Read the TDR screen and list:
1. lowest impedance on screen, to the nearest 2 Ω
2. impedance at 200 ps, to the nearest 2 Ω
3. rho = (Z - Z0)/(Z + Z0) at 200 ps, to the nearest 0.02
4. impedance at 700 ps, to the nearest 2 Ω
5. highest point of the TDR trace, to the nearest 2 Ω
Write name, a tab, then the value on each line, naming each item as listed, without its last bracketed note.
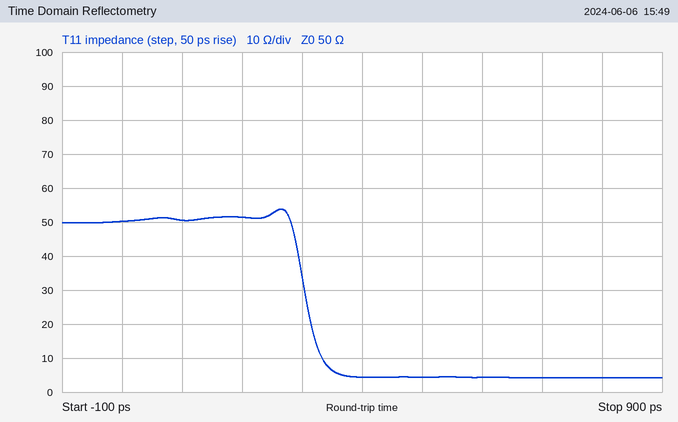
lowest impedance on screen, to the nearest 2 Ω	4 Ω
impedance at 200 ps, to the nearest 2 Ω	52 Ω
rho = (Z - Z0)/(Z + Z0) at 200 ps, to the nearest 0.02	+0.02
impedance at 700 ps, to the nearest 2 Ω	4 Ω
highest point of the TDR trace, to the nearest 2 Ω	54 Ω
